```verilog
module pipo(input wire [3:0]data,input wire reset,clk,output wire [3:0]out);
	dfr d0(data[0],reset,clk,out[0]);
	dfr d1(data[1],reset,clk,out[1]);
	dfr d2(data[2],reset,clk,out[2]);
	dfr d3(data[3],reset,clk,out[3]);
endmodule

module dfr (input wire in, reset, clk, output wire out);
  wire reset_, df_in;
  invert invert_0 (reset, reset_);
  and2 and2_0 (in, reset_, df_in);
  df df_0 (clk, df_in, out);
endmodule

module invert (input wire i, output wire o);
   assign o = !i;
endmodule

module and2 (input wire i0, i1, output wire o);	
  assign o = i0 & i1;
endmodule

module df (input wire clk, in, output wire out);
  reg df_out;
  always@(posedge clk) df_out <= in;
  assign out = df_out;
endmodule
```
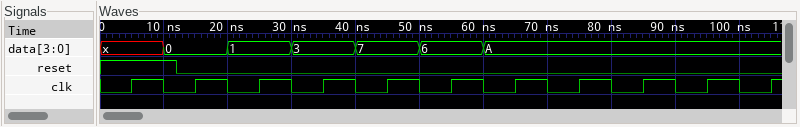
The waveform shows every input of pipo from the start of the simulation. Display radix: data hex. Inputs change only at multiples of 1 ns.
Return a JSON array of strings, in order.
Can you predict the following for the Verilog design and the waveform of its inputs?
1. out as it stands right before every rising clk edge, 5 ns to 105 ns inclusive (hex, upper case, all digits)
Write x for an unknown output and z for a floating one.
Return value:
["x, 0, 0, 1, 3, 7, 6, A, A, A, A"]
